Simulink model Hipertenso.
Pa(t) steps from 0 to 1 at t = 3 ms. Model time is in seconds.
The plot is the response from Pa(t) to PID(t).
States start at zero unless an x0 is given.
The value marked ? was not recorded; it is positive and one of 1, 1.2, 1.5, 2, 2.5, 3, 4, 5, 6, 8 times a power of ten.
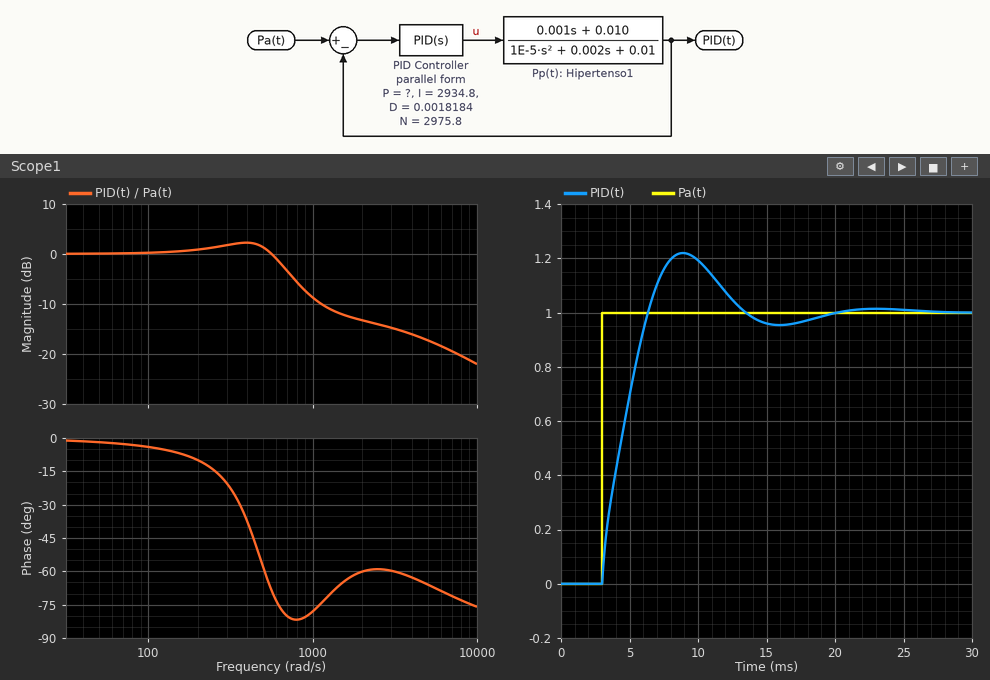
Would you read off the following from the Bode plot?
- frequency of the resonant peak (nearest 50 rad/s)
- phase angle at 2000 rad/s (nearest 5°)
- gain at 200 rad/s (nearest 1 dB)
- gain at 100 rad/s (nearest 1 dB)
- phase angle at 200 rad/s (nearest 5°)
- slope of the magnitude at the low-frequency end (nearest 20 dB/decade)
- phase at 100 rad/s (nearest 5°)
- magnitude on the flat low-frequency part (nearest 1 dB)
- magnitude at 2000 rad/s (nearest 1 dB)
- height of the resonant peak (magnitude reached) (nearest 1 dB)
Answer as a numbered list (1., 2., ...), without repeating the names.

1. 400 rad/s
2. -60°
3. 1 dB
4. 0 dB
5. -10°
6. 0 dB/decade
7. -5°
8. 0 dB
9. -13 dB
10. 2 dB
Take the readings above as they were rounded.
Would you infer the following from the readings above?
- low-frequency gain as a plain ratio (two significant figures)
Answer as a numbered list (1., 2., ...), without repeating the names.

1. 1.0
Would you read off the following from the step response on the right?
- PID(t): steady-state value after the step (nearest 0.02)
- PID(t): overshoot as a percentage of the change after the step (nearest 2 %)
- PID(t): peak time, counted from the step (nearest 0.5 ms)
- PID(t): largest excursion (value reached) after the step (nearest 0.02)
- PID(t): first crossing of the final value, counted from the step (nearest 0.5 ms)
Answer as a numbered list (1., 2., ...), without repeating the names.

1. 1.00
2. 22 %
3. 6.0 ms
4. 1.22
5. 3.5 ms
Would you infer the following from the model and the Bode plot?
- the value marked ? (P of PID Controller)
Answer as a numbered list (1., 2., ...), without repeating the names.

1. 3
